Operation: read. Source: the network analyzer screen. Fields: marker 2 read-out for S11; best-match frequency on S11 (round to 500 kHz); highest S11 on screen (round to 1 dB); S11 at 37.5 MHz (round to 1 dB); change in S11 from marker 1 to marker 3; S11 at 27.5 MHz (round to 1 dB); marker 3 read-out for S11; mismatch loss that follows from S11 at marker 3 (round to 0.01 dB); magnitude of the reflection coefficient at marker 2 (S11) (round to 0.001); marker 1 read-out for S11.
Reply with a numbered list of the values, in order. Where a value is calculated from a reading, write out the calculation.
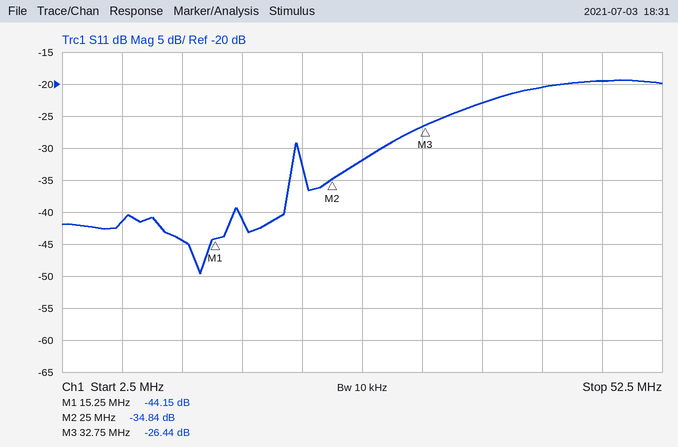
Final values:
1. -34.84 dB
2. 14.0 MHz
3. -19 dB
4. -23 dB
5. -26.44 − (-44.15) = 17.71 dB
6. -32 dB
7. -26.44 dB
8. −10 log10(1 − 10^(-26.44/10)) ≈ 0.01 dB
9. 10^(-34.84/20) ≈ 0.018
10. -44.15 dB
